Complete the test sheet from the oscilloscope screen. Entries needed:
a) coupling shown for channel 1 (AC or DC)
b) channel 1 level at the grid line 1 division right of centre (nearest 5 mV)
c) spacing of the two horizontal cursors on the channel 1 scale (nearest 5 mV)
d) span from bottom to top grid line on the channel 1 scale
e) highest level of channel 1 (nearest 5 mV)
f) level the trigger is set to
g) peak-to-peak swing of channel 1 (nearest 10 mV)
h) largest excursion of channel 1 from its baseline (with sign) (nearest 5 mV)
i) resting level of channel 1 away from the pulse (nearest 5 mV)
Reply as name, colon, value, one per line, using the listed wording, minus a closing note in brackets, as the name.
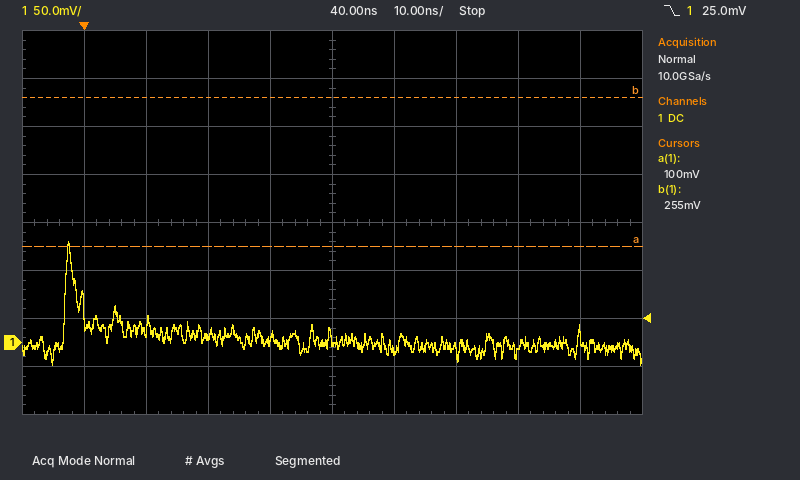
coupling shown for channel 1: DC
channel 1 level at the grid line 1 division right of centre: -10 mV
spacing of the two horizontal cursors on the channel 1 scale: 155 mV
span from bottom to top grid line on the channel 1 scale: 400 mV
highest level of channel 1: 105 mV
level the trigger is set to: 25.0 mV
peak-to-peak swing of channel 1: 130 mV
largest excursion of channel 1 from its baseline (with sign): +105 mV
resting level of channel 1 away from the pulse: 0 mV
